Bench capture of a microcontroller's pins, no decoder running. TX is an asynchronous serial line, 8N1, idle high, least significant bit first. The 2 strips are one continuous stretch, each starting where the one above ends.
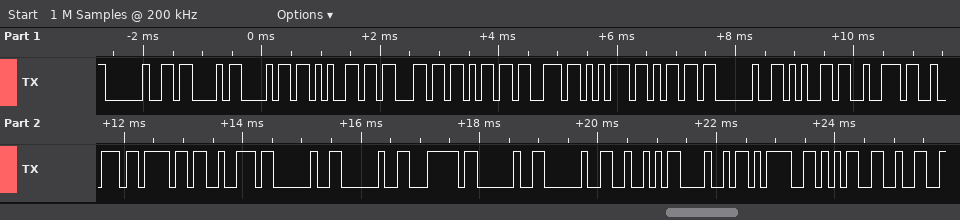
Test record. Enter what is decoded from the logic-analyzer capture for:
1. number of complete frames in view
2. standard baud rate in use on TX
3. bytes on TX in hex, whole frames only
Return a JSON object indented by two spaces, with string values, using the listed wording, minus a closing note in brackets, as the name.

{
  "number of complete frames in view": "25",
  "standard baud rate in use on TX": "9600 baud",
  "bytes on TX in hex, whole frames only": "20 43 68 65 63 6B 73 75 6D 20 65 72 72 6F 72 20 20 7C 20 20 52 48 3D 35 32"
}
